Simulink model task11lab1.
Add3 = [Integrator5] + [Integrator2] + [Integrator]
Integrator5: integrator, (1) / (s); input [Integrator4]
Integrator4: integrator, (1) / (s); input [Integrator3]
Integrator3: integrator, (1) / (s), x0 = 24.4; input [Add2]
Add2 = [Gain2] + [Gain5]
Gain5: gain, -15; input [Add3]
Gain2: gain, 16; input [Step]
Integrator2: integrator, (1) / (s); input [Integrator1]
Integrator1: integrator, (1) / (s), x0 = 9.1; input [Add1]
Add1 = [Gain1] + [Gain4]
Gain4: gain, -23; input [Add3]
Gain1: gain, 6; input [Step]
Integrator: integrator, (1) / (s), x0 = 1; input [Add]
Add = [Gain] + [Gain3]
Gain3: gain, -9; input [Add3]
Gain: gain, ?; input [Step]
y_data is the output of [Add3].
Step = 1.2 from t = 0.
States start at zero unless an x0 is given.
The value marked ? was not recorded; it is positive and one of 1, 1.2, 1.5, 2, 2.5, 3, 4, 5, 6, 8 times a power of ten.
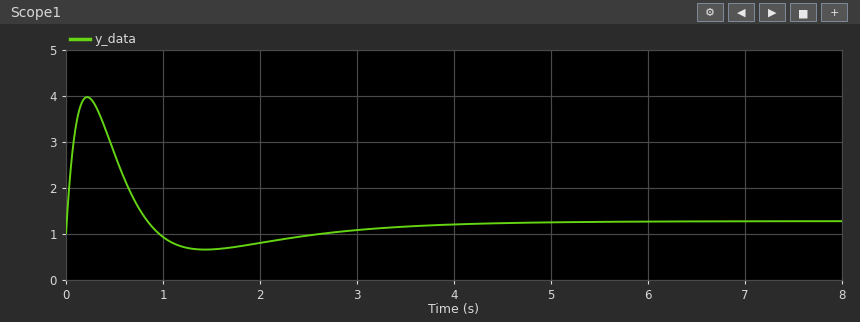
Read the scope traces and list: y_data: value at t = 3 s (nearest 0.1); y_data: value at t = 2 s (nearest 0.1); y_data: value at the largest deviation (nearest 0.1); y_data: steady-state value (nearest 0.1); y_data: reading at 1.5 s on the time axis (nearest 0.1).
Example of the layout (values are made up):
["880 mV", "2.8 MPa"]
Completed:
["1.1", "0.8", "4.0", "1.3", "0.7"]
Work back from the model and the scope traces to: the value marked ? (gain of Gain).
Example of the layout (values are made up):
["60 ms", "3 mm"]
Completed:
["30"]
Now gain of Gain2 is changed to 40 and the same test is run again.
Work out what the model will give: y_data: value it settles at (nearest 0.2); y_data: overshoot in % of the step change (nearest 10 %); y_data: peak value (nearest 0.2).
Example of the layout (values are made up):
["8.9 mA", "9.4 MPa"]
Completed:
["3.2", "40 %", "4.0"]
